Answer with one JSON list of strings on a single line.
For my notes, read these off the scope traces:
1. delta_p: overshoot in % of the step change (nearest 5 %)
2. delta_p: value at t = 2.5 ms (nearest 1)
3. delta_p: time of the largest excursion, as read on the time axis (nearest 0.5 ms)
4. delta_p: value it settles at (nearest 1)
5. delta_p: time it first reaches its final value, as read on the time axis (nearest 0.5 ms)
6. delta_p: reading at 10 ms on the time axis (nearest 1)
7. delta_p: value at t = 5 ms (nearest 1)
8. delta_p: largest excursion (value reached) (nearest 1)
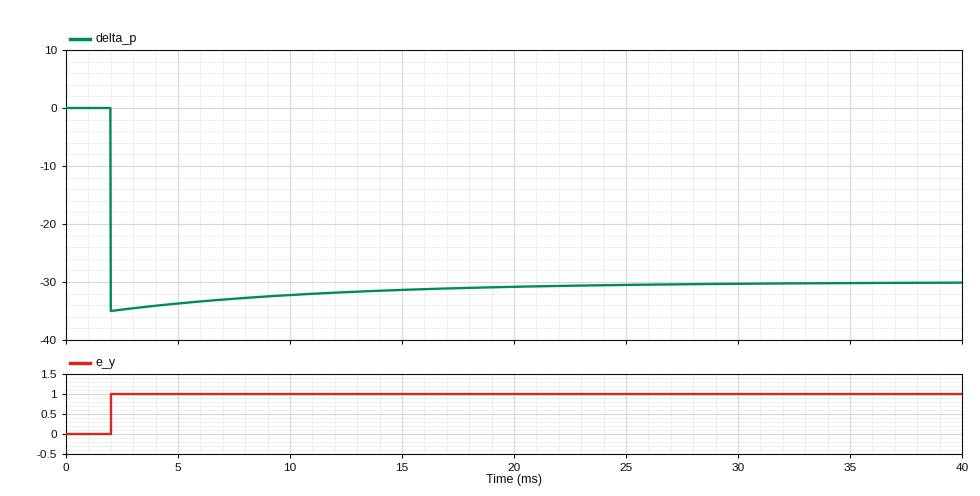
["15 %", "-35", "2.0 ms", "-30", "2.0 ms", "-32", "-34", "-35"]
